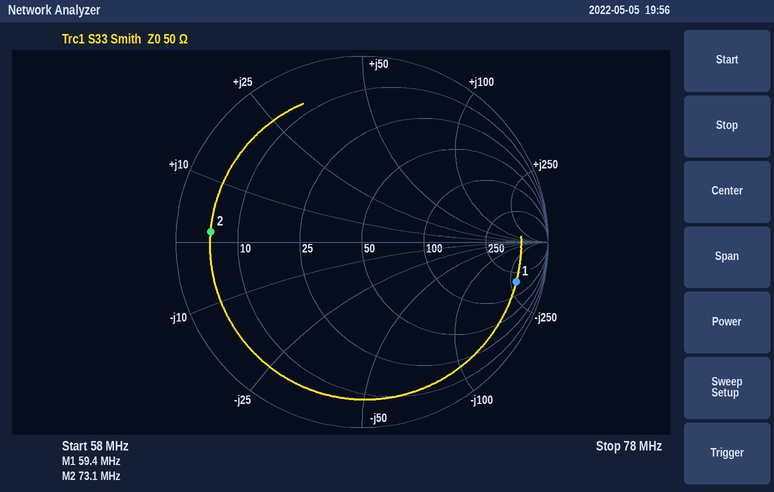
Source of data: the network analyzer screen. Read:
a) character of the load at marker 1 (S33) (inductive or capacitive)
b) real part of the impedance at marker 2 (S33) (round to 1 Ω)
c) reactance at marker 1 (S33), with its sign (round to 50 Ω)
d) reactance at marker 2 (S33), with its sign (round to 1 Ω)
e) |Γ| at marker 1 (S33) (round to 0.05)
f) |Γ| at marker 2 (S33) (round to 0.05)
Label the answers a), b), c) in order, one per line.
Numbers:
a) capacitive
b) 5 Ω
c) -300 Ω
d) +2 Ω
e) 0.85
f) 0.80
